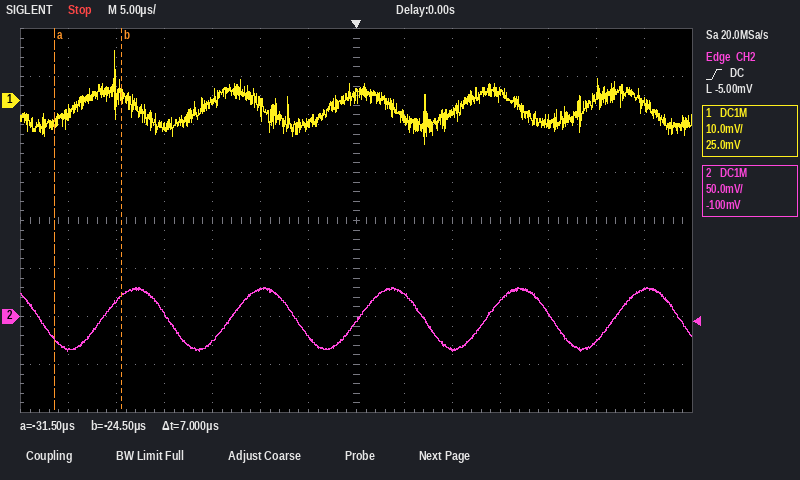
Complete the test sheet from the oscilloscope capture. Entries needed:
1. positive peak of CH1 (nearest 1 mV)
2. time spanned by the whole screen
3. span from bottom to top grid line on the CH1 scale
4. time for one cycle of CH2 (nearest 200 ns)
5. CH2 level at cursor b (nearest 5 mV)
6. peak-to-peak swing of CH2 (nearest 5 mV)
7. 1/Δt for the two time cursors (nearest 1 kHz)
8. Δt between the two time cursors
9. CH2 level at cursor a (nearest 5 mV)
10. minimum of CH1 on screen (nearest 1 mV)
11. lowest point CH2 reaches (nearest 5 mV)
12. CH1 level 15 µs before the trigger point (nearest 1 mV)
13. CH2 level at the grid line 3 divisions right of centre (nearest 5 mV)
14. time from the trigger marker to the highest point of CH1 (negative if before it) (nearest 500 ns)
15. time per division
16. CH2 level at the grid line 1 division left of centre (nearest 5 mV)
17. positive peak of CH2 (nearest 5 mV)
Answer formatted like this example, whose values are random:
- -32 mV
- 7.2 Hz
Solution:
- 10 mV
- 70 µs
- 80 mV
- 13.4 µs
- 20 mV
- 65 mV
- 143 kHz
- 7 µs
- -25 mV
- -9 mV
- -35 mV
- 0 mV
- 15 mV
- -25.0 µs
- 5 µs
- -20 mV
- 30 mV
